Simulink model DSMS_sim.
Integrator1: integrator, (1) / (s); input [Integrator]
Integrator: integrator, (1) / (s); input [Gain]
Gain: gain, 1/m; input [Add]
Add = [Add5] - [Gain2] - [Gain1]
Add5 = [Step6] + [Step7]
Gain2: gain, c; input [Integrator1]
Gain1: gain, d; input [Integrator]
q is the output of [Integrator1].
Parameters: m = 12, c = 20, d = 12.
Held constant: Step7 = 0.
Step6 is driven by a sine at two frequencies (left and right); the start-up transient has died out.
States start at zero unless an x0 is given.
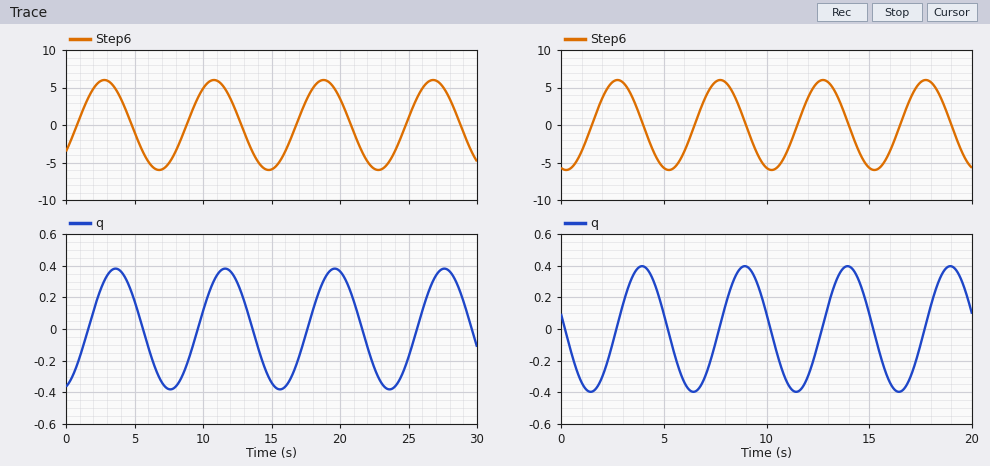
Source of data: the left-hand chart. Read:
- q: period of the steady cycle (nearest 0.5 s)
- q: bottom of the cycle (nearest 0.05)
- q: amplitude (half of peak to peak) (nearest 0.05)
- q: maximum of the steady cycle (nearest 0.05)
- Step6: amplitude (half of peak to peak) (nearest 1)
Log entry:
8.0 s
-0.40
0.40
0.40
6
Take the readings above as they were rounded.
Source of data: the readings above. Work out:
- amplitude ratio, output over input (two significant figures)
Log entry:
0.067
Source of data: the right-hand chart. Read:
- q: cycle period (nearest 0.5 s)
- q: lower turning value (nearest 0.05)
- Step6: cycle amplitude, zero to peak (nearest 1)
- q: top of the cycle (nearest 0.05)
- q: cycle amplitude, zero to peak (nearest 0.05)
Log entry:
5.0 s
-0.40
6
0.40
0.40
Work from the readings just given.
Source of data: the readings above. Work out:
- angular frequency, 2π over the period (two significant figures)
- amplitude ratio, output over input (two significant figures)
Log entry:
1.3 rad/s
0.067
